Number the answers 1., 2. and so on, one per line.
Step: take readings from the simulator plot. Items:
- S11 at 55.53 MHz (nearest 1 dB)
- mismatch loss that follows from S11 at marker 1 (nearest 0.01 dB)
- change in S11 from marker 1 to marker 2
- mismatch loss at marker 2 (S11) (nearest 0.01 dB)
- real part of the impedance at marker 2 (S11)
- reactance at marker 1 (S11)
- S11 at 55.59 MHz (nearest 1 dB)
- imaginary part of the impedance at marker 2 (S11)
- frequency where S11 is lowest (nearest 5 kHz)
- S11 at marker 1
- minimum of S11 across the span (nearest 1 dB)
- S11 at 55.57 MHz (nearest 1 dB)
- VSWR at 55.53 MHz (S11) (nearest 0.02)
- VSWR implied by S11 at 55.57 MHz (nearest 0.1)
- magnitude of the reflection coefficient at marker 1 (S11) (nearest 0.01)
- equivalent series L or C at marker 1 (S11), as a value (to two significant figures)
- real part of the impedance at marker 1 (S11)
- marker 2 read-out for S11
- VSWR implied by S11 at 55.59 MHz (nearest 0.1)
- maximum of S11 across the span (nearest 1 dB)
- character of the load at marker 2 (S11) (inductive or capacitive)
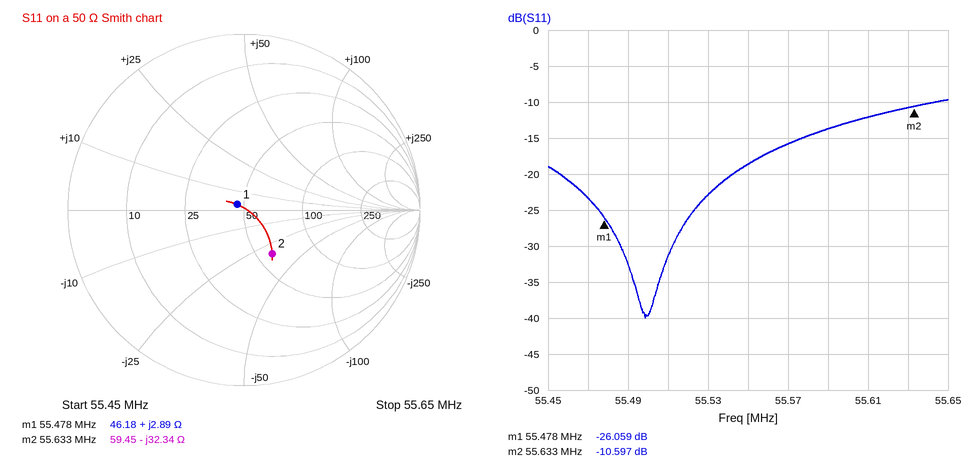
1. -23 dB
2. 0.01 dB
3. 15.462 dB
4. 0.40 dB
5. 59.45 Ω
6. +2.89 Ω
7. -14 dB
8. -32.34 Ω
9. 55.500 MHz
10. -26.059 dB
11. -40 dB
12. -16 dB
13. 1.16
14. 1.4
15. 0.05
16. 8.3 nH
17. 46.18 Ω
18. -10.597 dB
19. 1.5
20. -10 dB
21. capacitive
